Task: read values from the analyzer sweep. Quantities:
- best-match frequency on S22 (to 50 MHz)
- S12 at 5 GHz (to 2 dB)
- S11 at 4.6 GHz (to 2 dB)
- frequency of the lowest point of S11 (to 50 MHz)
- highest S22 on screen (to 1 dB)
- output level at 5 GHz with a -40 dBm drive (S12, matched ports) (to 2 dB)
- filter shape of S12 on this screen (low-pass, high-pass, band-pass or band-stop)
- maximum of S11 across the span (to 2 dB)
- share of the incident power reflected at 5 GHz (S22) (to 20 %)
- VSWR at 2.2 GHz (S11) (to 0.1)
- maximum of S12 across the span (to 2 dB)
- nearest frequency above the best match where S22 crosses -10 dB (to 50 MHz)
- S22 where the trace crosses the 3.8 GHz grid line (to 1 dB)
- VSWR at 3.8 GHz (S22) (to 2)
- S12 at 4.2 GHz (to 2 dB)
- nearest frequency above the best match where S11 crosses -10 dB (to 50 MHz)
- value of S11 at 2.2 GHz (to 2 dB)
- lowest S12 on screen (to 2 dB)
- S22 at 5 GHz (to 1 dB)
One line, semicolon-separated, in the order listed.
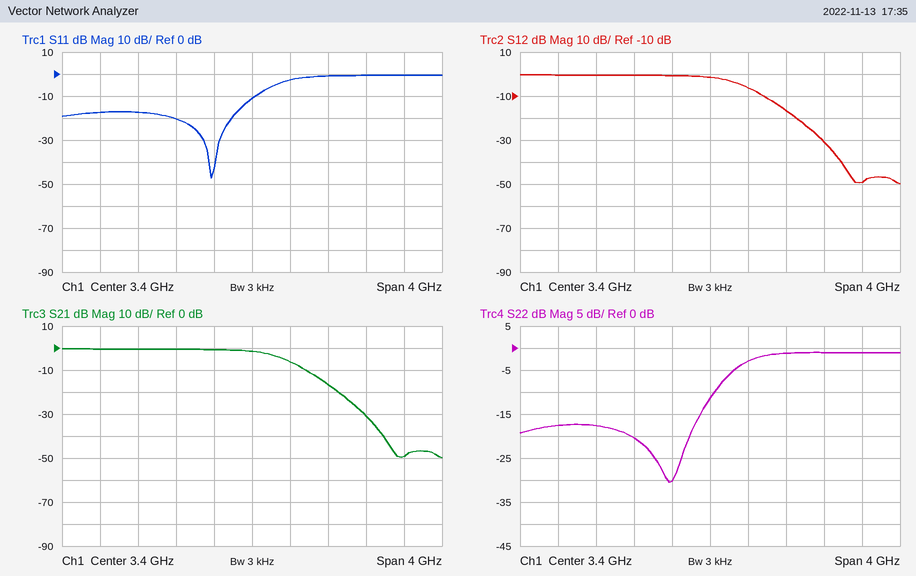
2.95 GHz; -50 dB; 0 dB; 2.95 GHz; -1 dB; -90 dBm; low-pass; 0 dB; 80 %; 1.3; 0 dB; 3.45 GHz; -3 dB; 6; -16 dB; 3.45 GHz; -18 dB; -50 dB; -1 dB
